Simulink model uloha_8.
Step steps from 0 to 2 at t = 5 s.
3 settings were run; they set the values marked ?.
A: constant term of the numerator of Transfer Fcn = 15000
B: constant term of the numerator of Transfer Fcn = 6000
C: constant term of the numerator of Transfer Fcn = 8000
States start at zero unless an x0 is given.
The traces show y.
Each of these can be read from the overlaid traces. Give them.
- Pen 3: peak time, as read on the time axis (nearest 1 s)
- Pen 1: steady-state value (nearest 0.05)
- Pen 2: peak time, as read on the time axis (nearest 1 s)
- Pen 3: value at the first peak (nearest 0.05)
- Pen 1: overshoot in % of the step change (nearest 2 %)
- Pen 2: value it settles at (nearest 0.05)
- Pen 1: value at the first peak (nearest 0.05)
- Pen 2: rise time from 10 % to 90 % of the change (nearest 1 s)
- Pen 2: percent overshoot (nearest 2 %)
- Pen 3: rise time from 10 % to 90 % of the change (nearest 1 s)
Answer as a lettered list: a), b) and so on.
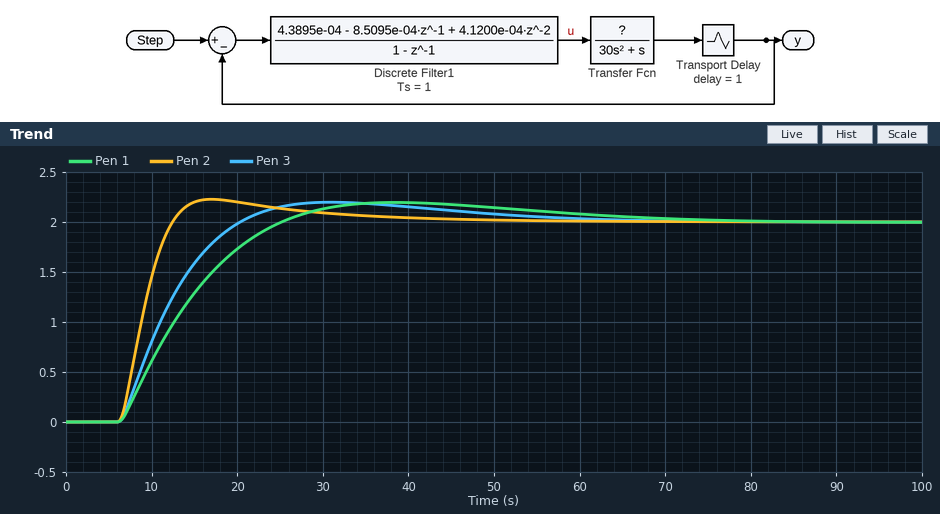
a) 31 s
b) 2.00
c) 17 s
d) 2.20
e) 10 %
f) 2.00
g) 2.20
h) 4 s
i) 12 %
j) 10 s
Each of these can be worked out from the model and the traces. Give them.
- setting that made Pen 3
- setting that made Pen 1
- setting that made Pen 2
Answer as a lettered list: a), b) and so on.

a) C
b) B
c) A
